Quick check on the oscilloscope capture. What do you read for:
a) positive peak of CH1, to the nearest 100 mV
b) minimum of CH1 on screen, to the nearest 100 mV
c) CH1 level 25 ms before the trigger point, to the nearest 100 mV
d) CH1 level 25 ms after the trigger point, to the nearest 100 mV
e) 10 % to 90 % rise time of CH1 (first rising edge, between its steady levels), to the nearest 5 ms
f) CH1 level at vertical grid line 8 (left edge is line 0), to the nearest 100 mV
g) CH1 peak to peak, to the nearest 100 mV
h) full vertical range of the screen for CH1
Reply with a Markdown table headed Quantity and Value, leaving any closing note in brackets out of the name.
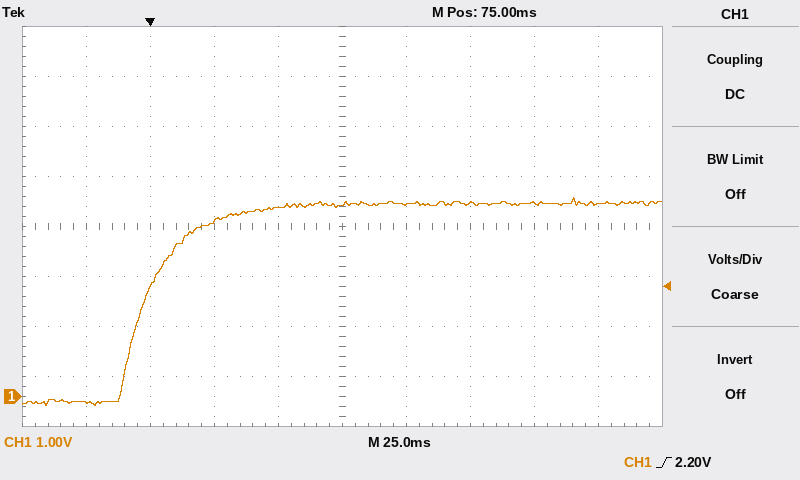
| Quantity | Value |
|---|---|
| positive peak of CH1, to the nearest 100 mV | 4.0 V |
| minimum of CH1 on screen, to the nearest 100 mV | -200 mV |
| CH1 level 25 ms before the trigger point, to the nearest 100 mV | -100 mV |
| CH1 level 25 ms after the trigger point, to the nearest 100 mV | 3.5 V |
| 10 % to 90 % rise time of CH1 (first rising edge, between its steady levels), to the nearest 5 ms | 35 ms |
| CH1 level at vertical grid line 8 (left edge is line 0), to the nearest 100 mV | 3.9 V |
| CH1 peak to peak, to the nearest 100 mV | 4.2 V |
| full vertical range of the screen for CH1 | 8 V |
